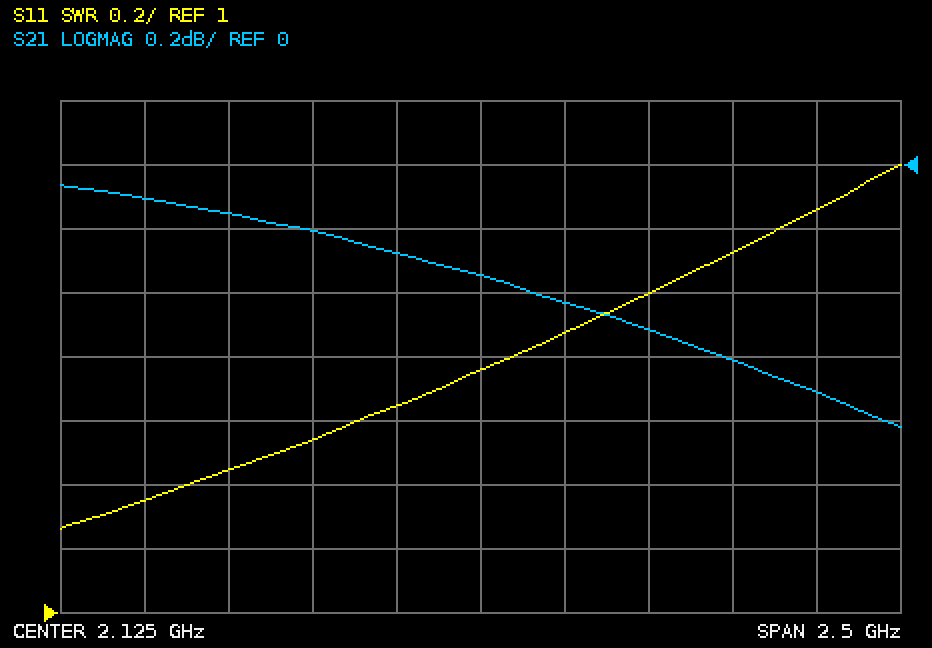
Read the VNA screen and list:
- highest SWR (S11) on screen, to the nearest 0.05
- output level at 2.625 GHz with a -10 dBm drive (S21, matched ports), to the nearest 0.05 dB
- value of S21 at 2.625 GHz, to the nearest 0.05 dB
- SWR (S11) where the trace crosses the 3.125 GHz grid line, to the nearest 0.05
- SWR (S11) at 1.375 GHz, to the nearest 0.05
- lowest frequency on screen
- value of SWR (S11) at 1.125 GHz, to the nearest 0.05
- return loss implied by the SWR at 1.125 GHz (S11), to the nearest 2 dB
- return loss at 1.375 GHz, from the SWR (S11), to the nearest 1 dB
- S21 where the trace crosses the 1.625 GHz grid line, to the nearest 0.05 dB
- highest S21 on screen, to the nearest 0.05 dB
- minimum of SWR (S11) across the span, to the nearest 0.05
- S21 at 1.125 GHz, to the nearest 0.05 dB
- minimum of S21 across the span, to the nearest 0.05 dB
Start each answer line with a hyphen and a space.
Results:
- 2.40
- -10.50 dBm
- -0.50 dB
- 2.25
- 1.45
- 875 MHz
- 1.35
- 16 dB
- 15 dB
- -0.20 dB
- -0.05 dB
- 1.25
- -0.10 dB
- -0.80 dB
